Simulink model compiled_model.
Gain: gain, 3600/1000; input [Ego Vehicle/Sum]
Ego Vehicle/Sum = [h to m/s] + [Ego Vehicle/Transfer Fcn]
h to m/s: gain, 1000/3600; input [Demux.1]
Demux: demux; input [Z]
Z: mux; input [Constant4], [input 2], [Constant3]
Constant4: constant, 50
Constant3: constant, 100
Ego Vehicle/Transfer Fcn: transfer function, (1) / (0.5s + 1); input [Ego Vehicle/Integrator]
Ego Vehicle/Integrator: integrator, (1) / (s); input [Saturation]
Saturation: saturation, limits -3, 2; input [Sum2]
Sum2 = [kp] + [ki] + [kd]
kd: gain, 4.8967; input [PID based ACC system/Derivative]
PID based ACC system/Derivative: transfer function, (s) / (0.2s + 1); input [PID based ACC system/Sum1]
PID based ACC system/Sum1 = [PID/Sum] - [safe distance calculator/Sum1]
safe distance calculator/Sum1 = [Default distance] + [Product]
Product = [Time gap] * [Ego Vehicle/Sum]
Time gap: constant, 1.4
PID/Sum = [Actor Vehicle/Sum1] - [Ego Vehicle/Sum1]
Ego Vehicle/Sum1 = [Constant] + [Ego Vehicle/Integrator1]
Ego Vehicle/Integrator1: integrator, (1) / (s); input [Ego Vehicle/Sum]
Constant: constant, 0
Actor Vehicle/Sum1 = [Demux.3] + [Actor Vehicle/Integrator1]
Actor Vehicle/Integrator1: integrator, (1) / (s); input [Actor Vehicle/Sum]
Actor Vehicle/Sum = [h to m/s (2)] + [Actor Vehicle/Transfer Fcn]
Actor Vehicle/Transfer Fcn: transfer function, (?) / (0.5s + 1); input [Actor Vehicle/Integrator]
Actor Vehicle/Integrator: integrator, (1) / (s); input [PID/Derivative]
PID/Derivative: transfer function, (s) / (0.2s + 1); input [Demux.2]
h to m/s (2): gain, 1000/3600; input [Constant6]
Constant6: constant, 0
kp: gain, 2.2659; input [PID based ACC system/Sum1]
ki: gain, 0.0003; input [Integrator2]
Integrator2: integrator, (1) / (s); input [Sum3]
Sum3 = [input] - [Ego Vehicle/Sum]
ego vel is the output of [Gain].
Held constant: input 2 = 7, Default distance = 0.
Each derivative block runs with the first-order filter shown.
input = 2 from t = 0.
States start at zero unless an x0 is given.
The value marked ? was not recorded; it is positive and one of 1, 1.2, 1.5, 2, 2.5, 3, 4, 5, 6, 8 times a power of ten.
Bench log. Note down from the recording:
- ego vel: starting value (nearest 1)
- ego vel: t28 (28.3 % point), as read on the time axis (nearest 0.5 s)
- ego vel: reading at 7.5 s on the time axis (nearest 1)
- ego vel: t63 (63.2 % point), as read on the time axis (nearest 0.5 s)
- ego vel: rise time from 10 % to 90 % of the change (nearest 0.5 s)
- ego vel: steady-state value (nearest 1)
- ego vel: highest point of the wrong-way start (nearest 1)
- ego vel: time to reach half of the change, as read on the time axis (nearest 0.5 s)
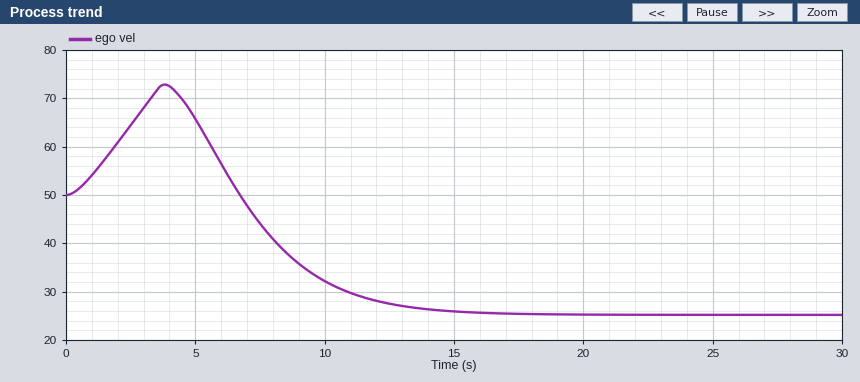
50
7.5 s
44
9.5 s
5.5 s
25
73
8.5 s
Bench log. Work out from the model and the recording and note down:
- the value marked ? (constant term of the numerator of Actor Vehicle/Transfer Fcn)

1
